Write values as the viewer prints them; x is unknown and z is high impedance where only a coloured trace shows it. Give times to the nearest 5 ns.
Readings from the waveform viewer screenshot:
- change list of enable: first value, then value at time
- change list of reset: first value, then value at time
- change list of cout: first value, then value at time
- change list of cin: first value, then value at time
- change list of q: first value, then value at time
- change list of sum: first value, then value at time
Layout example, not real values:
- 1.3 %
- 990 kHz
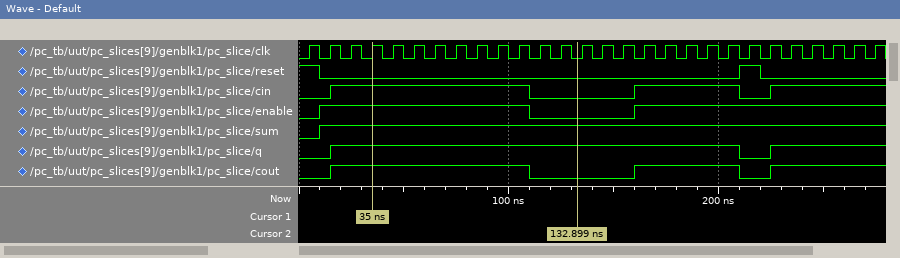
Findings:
- 0, 1 at 10 ns, 0 at 110 ns, 1 at 160 ns
- 1, 0 at 10 ns, 1 at 210 ns, 0 at 220 ns
- 0, 1 at 15 ns, 0 at 110 ns, 1 at 160 ns, 0 at 210 ns, 1 at 225 ns
- 0, 1 at 15 ns, 0 at 110 ns, 1 at 160 ns, 0 at 210 ns, 1 at 225 ns
- 0, 1 at 15 ns, 0 at 210 ns, 1 at 225 ns
- 0, 1 at 10 ns
